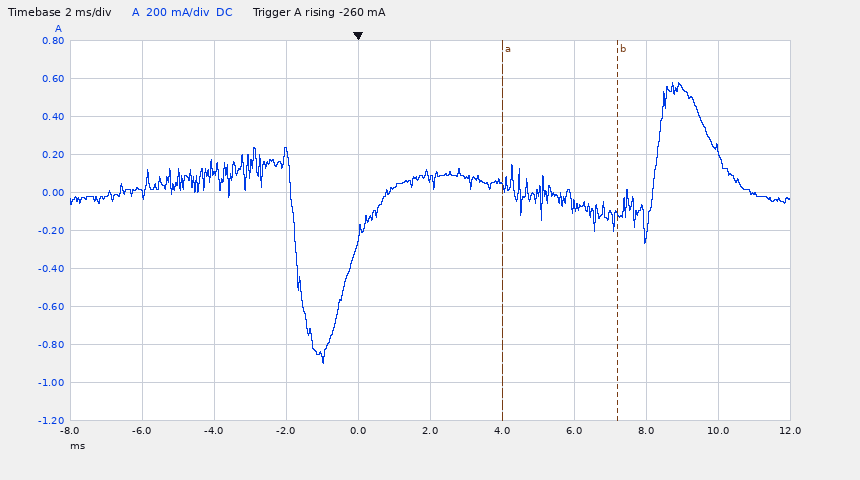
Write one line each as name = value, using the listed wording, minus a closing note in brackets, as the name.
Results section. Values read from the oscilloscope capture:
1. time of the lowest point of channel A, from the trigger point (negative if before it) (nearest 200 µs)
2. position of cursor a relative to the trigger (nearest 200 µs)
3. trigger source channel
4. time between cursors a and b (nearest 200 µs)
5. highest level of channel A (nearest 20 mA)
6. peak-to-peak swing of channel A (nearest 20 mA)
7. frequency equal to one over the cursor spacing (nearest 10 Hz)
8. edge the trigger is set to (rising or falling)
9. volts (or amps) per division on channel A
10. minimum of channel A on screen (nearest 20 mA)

time of the lowest point of channel A, from the trigger point (negative if before it) = -1.0 ms
position of cursor a relative to the trigger = +4.0 ms
trigger source channel = channel A
time between cursors a and b = 3.2 ms
highest level of channel A = 580 mA
peak-to-peak swing of channel A = 1.48 A
frequency equal to one over the cursor spacing = 310 Hz
edge the trigger is set to = rising
volts (or amps) per division on channel A = 200 mA
minimum of channel A on screen = -900 mA
